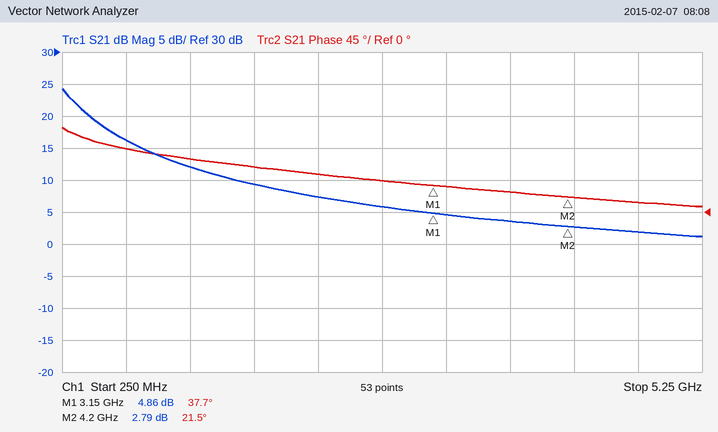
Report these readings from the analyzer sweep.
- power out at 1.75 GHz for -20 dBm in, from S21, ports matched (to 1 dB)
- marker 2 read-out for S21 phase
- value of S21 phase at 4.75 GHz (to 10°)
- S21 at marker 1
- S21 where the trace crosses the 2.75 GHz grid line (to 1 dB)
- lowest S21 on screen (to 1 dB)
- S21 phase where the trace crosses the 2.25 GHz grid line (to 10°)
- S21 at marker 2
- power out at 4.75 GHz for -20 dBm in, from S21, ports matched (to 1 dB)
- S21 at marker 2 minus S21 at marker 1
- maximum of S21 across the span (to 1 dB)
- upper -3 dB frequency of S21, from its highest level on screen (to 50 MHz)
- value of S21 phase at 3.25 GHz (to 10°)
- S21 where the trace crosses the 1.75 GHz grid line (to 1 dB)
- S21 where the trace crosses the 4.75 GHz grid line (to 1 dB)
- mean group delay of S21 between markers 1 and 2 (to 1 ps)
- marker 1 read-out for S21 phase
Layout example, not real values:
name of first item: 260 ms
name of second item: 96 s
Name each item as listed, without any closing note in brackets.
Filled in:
power out at 1.75 GHz for -20 dBm in, from S21, ports matched: -11 dBm
marker 2 read-out for S21 phase: 21.5°
value of S21 phase at 4.75 GHz: 10°
S21 at marker 1: 4.86 dB
S21 where the trace crosses the 2.75 GHz grid line: 6 dB
lowest S21 on screen: 1 dB
S21 phase where the trace crosses the 2.25 GHz grid line: 50°
S21 at marker 2: 2.79 dB
power out at 4.75 GHz for -20 dBm in, from S21, ports matched: -18 dBm
S21 at marker 2 minus S21 at marker 1: -2.07 dB
maximum of S21 across the span: 24 dB
upper -3 dB frequency of S21, from its highest level on screen: 400 MHz
value of S21 phase at 3.25 GHz: 40°
S21 where the trace crosses the 1.75 GHz grid line: 9 dB
S21 where the trace crosses the 4.75 GHz grid line: 2 dB
mean group delay of S21 between markers 1 and 2: 43 ps
marker 1 read-out for S21 phase: 37.7°
